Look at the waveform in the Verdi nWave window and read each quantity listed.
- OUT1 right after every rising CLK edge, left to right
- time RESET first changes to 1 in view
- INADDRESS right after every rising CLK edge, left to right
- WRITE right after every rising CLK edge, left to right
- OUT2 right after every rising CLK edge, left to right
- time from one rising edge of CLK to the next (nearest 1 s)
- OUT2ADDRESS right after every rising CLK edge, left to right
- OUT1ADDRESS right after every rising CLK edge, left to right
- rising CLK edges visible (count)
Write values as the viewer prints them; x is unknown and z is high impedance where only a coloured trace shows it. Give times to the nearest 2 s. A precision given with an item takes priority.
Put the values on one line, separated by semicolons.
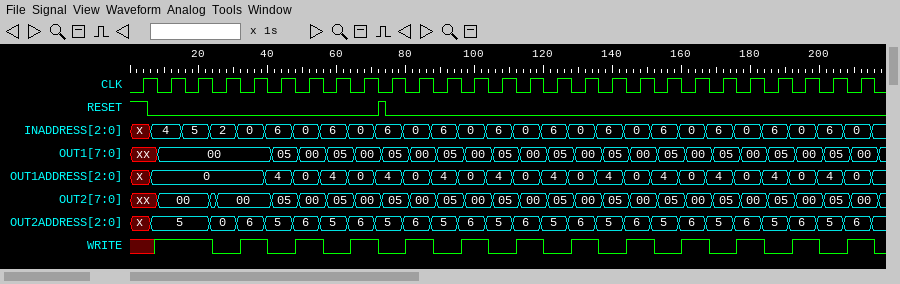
xx, 00, 00, 00, 00, 05, 00, 05, 00, 05, 00, 05, 00, 05, 00, 05, 00, 05, 00, 05, 00, 05, 00, 05, 00, 05, 00; 72 s; x, 4, 5, 2, 0, 6, 0, 6, 0, 6, 0, 6, 0, 6, 0, 6, 0, 6, 0, 6, 0, 6, 0, 6, 0, 6, 0; x 1 1 0 1 0 1 0 1 0 1 0 1 0 1 0 1 0 1 0 1 0 1 0 1 0 1; xx, 00, 00, 00, 00, 05, 00, 05, 00, 05, 00, 05, 00, 05, 00, 05, 00, 05, 00, 05, 00, 05, 00, 05, 00, 05, 00; 8 s; x, 5, 5, 0, 6, 5, 6, 5, 6, 5, 6, 5, 6, 5, 6, 5, 6, 5, 6, 5, 6, 5, 6, 5, 6, 5, 6; x, 0, 0, 0, 0, 4, 0, 4, 0, 4, 0, 4, 0, 4, 0, 4, 0, 4, 0, 4, 0, 4, 0, 4, 0, 4, 0; 27
